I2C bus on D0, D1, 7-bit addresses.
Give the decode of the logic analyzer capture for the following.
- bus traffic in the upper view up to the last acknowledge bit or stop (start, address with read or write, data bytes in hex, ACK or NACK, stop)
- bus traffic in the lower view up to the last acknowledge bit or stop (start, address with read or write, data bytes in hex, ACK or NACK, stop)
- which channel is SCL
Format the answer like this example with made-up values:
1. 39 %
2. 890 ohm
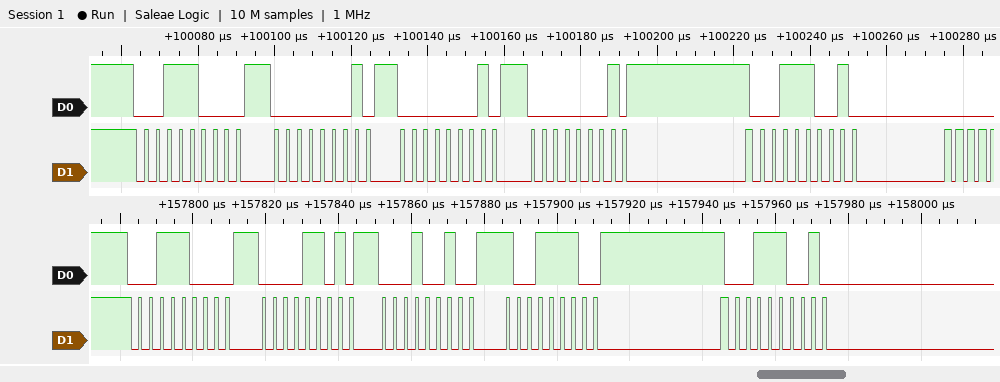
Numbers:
1. start, address 1C write ACK, 01 ACK, 01 ACK, 01 ACK, repeated start, address 1C read ACK
2. start, address 1C write ACK, 0D ACK, 12 ACK, 9E ACK, repeated start, address 1C read ACK
3. D1
